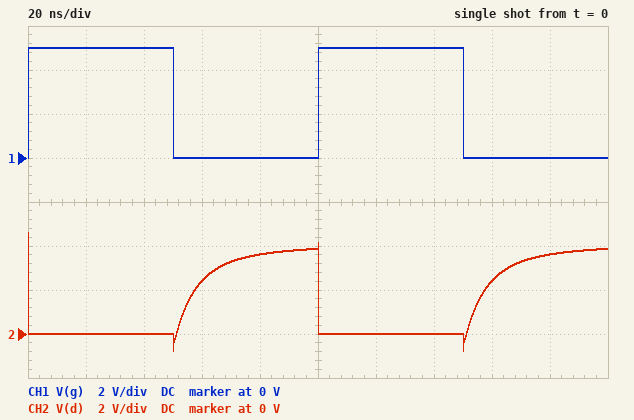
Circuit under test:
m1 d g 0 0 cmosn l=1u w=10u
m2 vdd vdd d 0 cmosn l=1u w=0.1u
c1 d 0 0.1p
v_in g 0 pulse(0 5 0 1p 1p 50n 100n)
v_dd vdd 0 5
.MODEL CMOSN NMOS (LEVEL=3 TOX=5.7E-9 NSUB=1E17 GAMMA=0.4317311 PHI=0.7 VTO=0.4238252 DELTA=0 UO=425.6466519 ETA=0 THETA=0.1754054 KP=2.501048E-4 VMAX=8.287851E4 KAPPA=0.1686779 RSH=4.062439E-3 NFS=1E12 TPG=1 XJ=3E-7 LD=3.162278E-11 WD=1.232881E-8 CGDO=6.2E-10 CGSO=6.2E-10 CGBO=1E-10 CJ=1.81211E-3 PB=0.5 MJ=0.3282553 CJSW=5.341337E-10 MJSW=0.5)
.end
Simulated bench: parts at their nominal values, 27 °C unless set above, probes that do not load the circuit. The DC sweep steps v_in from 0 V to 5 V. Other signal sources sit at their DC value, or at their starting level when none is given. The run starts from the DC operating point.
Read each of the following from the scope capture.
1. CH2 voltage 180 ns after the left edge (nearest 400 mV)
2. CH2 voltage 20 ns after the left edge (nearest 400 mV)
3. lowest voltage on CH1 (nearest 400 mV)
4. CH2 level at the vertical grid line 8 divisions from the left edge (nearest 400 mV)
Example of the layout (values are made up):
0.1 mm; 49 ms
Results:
3.6 V; 0 V; 0 V; 2.4 V
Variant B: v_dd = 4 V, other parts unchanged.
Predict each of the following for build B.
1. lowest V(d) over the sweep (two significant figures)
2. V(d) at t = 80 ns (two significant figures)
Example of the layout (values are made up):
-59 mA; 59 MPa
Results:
5.8 mV; 2.7 V
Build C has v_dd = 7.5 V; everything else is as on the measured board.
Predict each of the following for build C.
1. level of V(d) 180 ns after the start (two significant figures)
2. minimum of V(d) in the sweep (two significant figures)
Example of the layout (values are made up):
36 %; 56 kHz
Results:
5.9 V; 14 mV
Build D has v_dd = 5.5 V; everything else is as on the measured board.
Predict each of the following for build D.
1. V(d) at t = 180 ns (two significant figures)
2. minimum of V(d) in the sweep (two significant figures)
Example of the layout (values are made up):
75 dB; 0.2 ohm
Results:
4.1 V; 9.2 mV
